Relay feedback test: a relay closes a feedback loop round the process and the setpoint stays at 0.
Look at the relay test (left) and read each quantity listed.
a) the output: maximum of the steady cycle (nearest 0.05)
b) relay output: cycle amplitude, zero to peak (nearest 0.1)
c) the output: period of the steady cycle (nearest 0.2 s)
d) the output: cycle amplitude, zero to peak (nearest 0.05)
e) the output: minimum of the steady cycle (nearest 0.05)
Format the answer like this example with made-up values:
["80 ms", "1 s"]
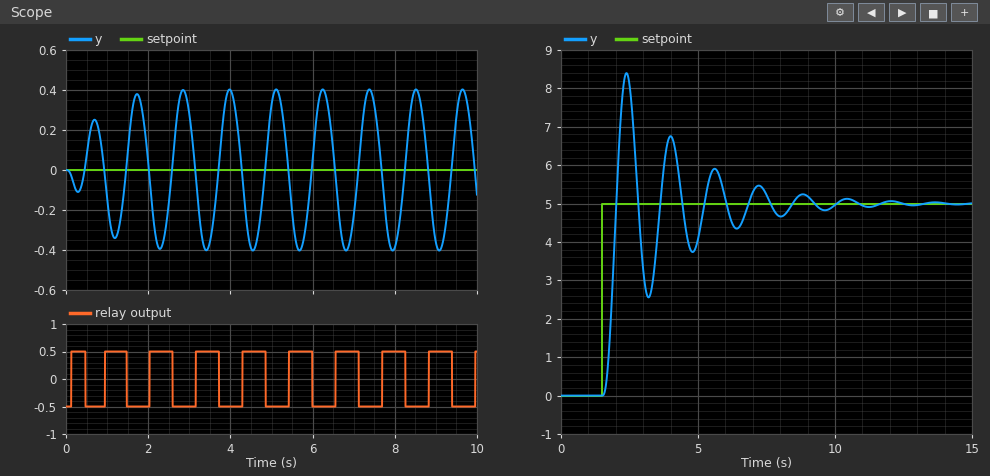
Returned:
["0.40", "0.5", "1.2 s", "0.40", "-0.40"]
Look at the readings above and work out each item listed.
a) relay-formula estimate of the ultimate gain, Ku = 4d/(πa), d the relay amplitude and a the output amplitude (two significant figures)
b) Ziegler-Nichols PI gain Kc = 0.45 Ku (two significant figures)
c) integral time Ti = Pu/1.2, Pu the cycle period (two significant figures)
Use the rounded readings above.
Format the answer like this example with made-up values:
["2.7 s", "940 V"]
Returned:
["1.6", "0.72", "1.0 s"]
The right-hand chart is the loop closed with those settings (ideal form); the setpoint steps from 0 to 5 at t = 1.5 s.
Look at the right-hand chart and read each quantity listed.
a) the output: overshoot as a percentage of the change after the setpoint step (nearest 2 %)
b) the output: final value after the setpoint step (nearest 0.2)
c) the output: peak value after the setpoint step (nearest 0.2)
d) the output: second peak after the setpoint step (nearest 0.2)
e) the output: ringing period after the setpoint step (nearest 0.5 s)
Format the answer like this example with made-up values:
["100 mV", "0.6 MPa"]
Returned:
["68 %", "5.0", "8.4", "6.8", "1.5 s"]
